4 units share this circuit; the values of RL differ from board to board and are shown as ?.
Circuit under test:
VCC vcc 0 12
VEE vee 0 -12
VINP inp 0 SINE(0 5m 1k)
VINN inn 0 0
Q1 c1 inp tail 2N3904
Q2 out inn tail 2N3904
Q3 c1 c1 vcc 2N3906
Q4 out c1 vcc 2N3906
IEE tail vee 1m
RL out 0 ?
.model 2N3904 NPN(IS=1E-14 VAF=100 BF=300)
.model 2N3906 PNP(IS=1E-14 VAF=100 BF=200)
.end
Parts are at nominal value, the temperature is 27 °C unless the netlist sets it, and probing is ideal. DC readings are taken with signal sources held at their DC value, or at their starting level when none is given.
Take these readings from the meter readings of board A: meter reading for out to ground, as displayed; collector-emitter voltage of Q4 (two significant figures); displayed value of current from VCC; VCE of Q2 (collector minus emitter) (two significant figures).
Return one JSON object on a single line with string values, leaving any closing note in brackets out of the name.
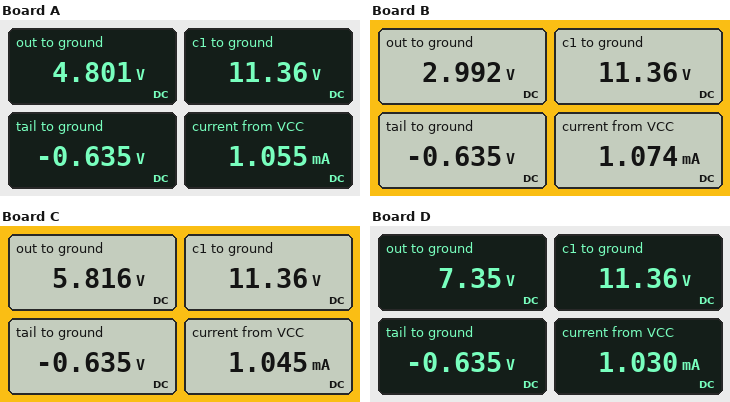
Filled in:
{"meter reading for out to ground, as displayed": "4.801 V", "collector-emitter voltage of Q4": "-7.2 V", "displayed value of current from VCC": "1.055 mA", "VCE of Q2 (collector minus emitter)": "5.4 V"}
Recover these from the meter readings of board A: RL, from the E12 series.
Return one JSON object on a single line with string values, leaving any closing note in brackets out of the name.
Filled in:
{"RL, from the E12 series": "82 kΩ"}
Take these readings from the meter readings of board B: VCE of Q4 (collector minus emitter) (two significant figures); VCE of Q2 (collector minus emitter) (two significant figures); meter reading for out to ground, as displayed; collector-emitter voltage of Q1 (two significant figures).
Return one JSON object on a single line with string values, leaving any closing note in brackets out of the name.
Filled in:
{"VCE of Q4 (collector minus emitter)": "-9.0 V", "VCE of Q2 (collector minus emitter)": "3.6 V", "meter reading for out to ground, as displayed": "2.992 V", "collector-emitter voltage of Q1": "12 V"}
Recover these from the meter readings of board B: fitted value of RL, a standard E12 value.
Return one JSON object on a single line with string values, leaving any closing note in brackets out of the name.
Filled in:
{"fitted value of RL, a standard E12 value": "39 kΩ"}
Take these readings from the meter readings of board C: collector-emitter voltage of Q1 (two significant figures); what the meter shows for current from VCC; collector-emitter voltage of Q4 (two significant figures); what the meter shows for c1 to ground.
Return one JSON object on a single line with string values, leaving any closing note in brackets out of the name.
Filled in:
{"collector-emitter voltage of Q1": "12 V", "what the meter shows for current from VCC": "1.045 mA", "collector-emitter voltage of Q4": "-6.2 V", "what the meter shows for c1 to ground": "11.36 V"}
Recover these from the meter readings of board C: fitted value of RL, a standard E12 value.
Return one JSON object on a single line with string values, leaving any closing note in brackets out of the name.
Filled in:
{"fitted value of RL, a standard E12 value": "120 kΩ"}
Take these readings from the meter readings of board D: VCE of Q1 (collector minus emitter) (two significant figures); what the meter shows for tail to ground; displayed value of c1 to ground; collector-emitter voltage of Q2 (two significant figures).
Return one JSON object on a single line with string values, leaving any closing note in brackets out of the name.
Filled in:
{"VCE of Q1 (collector minus emitter)": "12 V", "what the meter shows for tail to ground": "-0.635 V", "displayed value of c1 to ground": "11.36 V", "collector-emitter voltage of Q2": "8.0 V"}
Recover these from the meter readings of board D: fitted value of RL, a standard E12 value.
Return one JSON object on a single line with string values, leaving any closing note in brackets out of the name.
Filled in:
{"fitted value of RL, a standard E12 value": "220 kΩ"}
